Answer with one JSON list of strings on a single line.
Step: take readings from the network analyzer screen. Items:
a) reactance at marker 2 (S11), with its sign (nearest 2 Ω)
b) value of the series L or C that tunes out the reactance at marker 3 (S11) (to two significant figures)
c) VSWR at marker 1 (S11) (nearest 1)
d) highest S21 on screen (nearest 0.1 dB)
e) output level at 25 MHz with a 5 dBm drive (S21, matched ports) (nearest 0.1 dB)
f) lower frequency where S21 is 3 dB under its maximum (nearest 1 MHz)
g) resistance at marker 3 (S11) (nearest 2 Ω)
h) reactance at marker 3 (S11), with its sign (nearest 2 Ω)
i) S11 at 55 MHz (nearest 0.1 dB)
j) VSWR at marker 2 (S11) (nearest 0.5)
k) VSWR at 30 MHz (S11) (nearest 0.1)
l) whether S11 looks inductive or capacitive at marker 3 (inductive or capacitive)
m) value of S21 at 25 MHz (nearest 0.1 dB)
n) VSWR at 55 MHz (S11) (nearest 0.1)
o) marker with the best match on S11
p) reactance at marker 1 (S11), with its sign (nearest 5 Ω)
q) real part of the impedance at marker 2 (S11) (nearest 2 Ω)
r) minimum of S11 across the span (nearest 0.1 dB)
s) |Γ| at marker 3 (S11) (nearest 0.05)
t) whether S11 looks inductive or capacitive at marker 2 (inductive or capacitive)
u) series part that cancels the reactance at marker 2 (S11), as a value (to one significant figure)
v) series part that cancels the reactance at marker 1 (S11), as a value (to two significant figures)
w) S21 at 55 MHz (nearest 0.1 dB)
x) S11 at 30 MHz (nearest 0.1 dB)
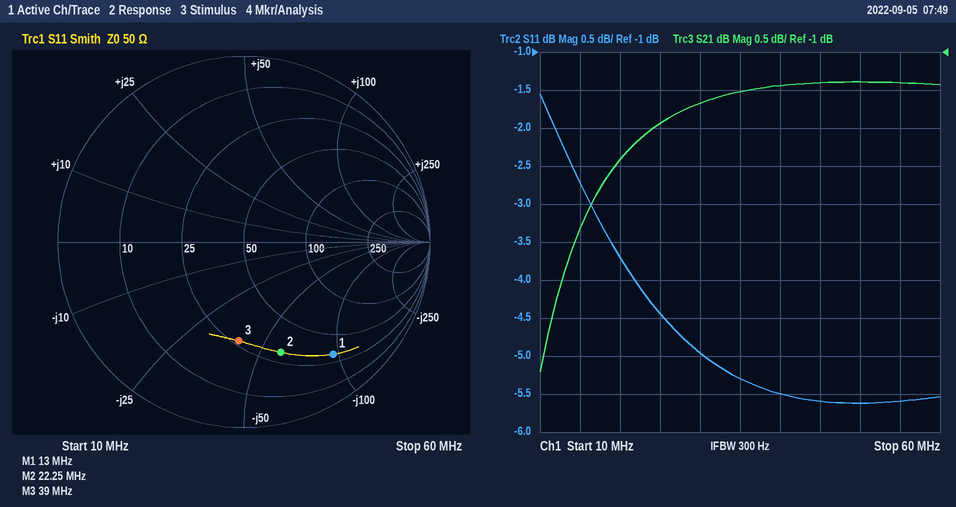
["-60 Ω", "160 nH", "8", "-1.4 dB", "3.1 dBm", "12 MHz", "26 Ω", "-40 Ω", "-5.6 dB", "4.5", "3.6", "capacitive", "-1.9 dB", "3.2", "marker 3", "-95 Ω", "30 Ω", "-5.6 dB", "0.55", "capacitive", "400 nH", "1.2 µH", "-1.4 dB", "-5.0 dB"]
